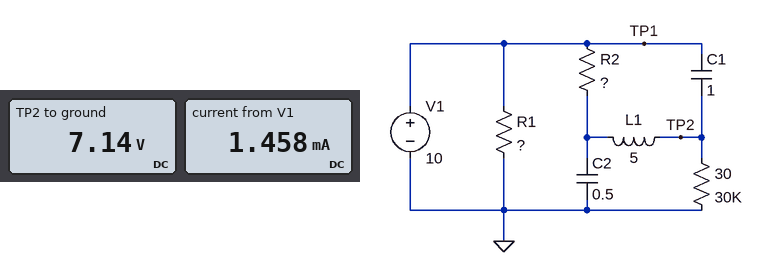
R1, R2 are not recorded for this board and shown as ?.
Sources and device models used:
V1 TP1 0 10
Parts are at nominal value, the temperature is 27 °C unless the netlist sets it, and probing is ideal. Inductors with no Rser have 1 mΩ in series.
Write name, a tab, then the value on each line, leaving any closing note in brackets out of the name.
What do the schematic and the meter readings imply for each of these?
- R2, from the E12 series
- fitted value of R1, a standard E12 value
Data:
R2, from the E12 series	12 kΩ
fitted value of R1, a standard E12 value	8.2 kΩ
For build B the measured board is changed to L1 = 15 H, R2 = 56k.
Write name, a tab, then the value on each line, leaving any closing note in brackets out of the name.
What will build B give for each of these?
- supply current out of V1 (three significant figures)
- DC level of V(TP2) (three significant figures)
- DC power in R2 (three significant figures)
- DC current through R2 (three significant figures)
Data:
supply current out of V1	1.34 mA
DC level of V(TP2)	3.49 V
DC power in R2	757 µW
DC current through R2	116 µA
